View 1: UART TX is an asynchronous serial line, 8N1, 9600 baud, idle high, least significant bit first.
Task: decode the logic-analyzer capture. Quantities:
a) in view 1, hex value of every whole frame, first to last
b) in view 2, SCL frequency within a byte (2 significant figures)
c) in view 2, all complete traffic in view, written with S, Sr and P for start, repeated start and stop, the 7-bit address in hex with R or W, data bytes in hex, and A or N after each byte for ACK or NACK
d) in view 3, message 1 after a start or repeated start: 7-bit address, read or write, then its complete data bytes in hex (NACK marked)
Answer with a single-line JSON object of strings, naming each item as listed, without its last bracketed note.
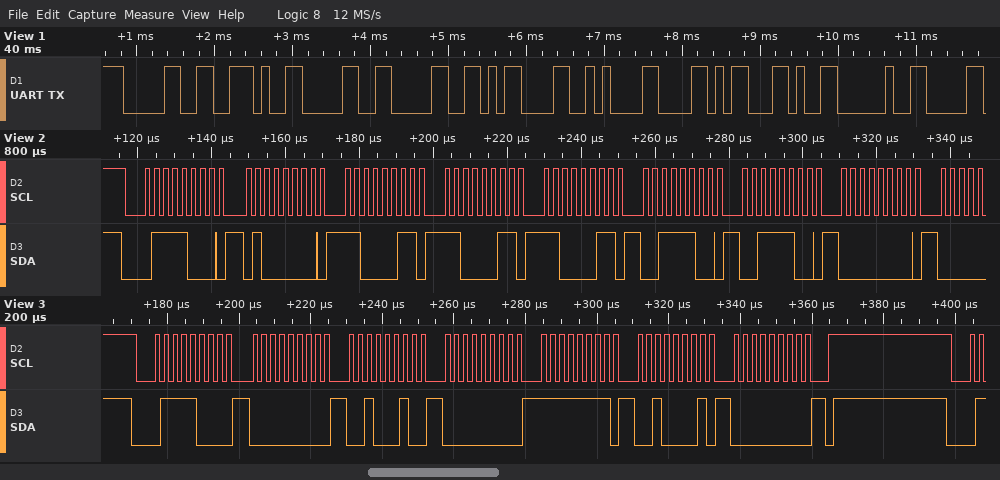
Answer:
{"in view 1, hex value of every whole frame, first to last": "30 2E 30 30 0D 0A 58 2C 20", "in view 2, SCL frequency within a byte": "400 kHz", "in view 2, all complete traffic in view, written with S, Sr and P for start, repeated start and stop, the 7-bit address in hex with R or W, data bytes in hex, and A or N after each byte for ACK or NACK": "S 3CW A 40 A C3 A C3 A C3 A 3C A 3C A 00 A", "in view 3, message 1 after a start or repeated start: 7-bit address, read or write, then its complete data bytes in hex": "0x3C write: 00 22 00 FF 21 00"}
